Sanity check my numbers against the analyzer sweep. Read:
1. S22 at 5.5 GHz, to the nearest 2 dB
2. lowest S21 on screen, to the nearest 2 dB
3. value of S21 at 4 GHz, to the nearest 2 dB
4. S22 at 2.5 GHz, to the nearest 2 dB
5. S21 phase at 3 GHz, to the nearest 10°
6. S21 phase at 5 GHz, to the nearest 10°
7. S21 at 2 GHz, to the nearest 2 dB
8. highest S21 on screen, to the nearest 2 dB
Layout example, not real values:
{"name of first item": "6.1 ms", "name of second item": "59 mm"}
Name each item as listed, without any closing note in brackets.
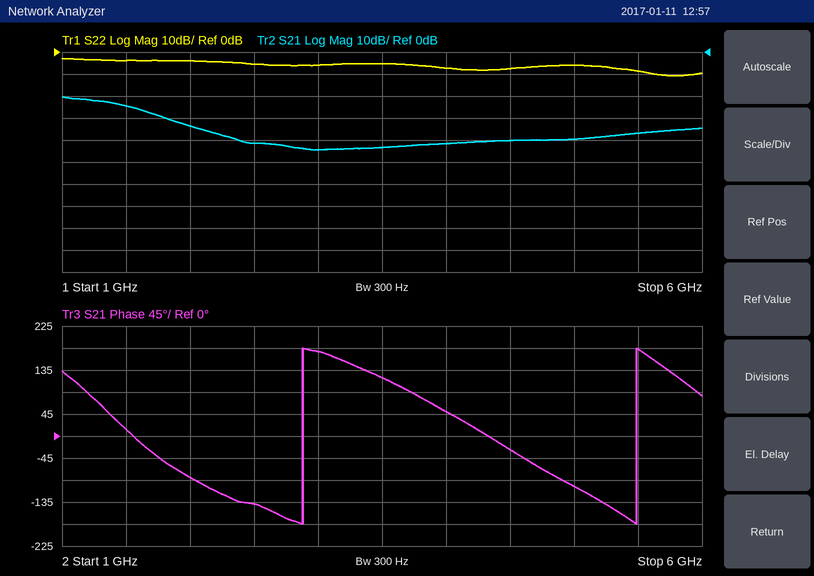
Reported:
{"S22 at 5.5 GHz, to the nearest 2 dB": "-8 dB", "lowest S21 on screen, to the nearest 2 dB": "-44 dB", "value of S21 at 4 GHz, to the nearest 2 dB": "-42 dB", "S22 at 2.5 GHz, to the nearest 2 dB": "-6 dB", "S21 phase at 3 GHz, to the nearest 10°": "170°", "S21 phase at 5 GHz, to the nearest 10°": "-100°", "S21 at 2 GHz, to the nearest 2 dB": "-34 dB", "highest S21 on screen, to the nearest 2 dB": "-20 dB"}
